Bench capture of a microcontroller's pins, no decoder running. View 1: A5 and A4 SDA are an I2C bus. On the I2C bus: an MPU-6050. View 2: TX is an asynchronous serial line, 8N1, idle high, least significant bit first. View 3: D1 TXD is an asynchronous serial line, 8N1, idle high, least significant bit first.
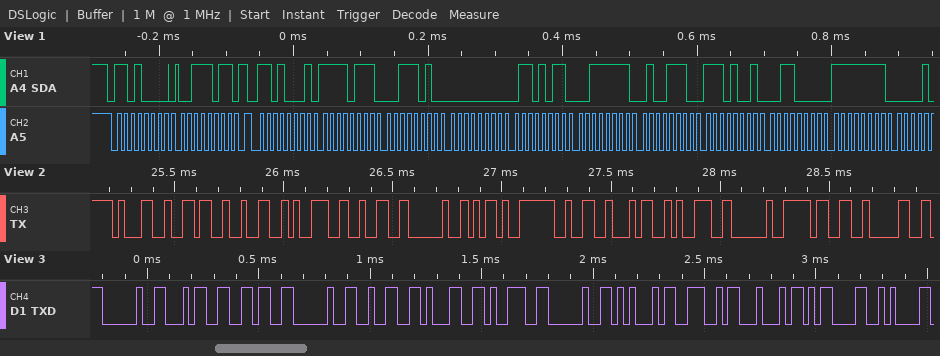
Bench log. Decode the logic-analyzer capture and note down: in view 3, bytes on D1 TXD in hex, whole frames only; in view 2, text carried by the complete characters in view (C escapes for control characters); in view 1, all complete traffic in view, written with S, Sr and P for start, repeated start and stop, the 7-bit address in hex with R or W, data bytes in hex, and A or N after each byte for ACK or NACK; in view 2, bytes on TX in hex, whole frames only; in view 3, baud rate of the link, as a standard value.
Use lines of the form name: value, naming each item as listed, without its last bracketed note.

in view 3, bytes on D1 TXD in hex, whole frames only: 20 34 36 20 32 31 39 20 45 4E 44 0D 0A
in view 2, text carried by the complete characters in view: "16292 -249 30"
in view 1, all complete traffic in view, written with S, Sr and P for start, repeated start and stop, the 7-bit address in hex with R or W, data bytes in hex, and A or N after each byte for ACK or NACK: S 68W A 3B A Sr 68R A F7 A 3A A 00 A 6B A 3F A 4E A E9 A 30 A FF A
in view 2, bytes on TX in hex, whole frames only: 31 36 32 39 32 20 2D 32 34 39 20 33 30
in view 3, baud rate of the link, as a standard value: 38400 baud
